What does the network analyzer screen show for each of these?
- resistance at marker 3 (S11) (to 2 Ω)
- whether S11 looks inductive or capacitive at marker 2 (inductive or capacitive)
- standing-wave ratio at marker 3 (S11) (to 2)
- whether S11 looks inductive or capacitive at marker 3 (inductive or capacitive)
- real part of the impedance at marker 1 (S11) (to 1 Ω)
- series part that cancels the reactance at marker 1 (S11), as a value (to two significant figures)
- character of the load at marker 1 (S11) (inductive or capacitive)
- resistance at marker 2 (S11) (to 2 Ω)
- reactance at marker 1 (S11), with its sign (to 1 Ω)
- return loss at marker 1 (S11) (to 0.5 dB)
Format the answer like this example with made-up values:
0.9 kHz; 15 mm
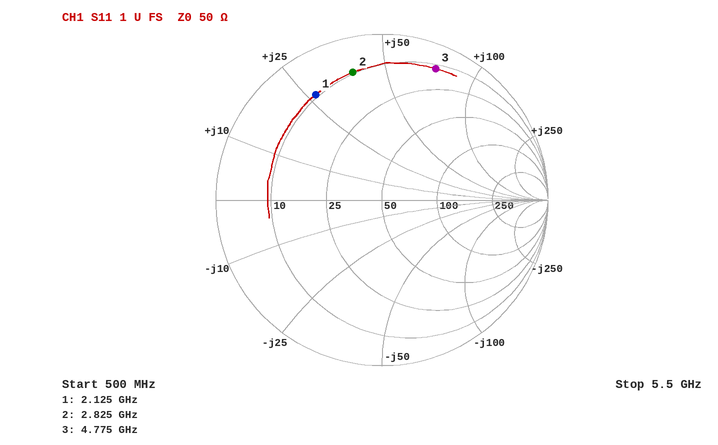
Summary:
12 Ω; inductive; 12; inductive; 9 Ω; 2.8 pF; inductive; 10 Ω; +27 Ω; 2.5 dB
